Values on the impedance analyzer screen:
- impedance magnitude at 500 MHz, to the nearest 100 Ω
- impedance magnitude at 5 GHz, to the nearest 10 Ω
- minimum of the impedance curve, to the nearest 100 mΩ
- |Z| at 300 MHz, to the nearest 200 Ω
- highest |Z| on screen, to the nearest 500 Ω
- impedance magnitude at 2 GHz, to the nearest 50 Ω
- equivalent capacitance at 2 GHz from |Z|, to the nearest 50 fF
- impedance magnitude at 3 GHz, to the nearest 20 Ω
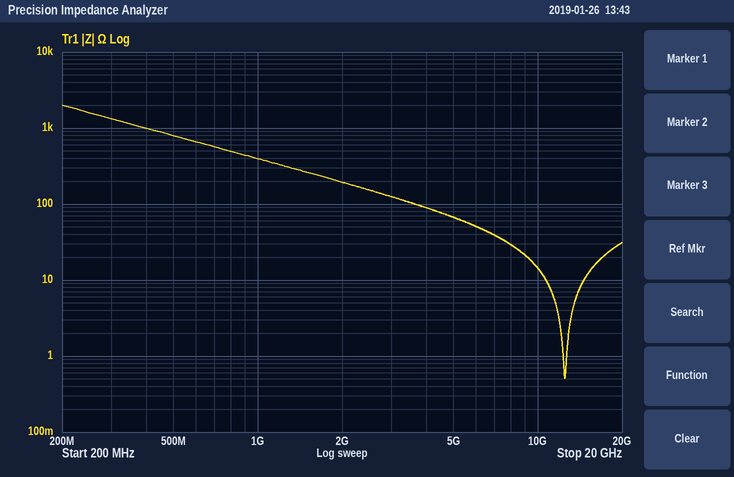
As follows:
800 Ω
70 Ω
500 mΩ
1.4 kΩ
2.0 kΩ
200 Ω
400 fF
120 Ω
